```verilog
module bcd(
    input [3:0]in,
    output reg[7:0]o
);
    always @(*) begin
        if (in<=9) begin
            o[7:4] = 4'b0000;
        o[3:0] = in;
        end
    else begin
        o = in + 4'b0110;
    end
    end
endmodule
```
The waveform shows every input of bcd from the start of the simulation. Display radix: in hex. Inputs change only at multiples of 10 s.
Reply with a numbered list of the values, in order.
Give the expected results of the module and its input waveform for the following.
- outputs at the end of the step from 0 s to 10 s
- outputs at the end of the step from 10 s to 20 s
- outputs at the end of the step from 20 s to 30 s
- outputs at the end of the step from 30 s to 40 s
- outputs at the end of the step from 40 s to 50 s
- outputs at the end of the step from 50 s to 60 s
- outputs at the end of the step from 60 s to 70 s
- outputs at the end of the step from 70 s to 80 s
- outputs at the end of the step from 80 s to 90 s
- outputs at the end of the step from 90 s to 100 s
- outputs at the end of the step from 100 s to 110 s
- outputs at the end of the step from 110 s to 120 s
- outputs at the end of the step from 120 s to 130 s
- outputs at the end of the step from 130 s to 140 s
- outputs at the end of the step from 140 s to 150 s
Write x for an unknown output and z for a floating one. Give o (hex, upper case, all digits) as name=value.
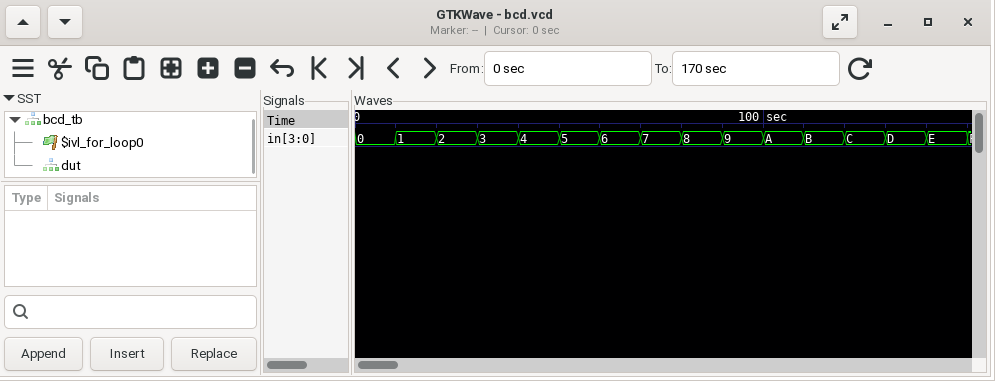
1. o=00
2. o=01
3. o=02
4. o=03
5. o=04
6. o=05
7. o=06
8. o=07
9. o=08
10. o=09
11. o=10
12. o=11
13. o=12
14. o=13
15. o=14
